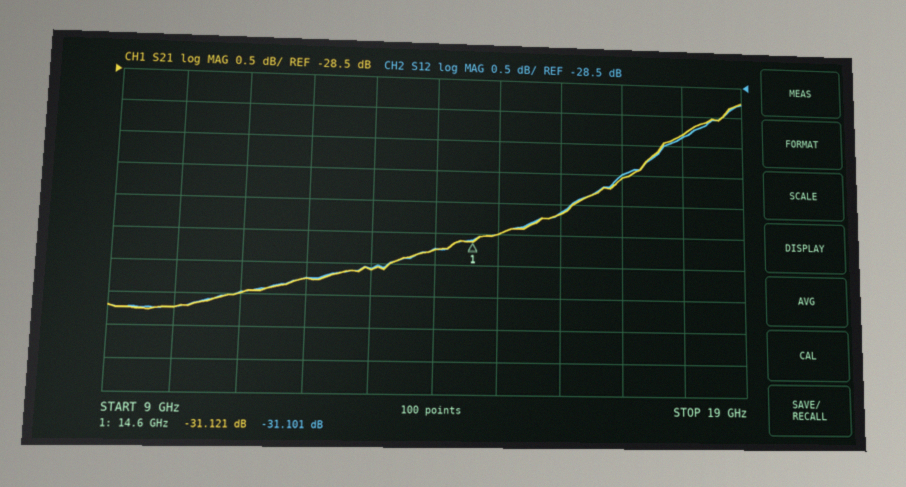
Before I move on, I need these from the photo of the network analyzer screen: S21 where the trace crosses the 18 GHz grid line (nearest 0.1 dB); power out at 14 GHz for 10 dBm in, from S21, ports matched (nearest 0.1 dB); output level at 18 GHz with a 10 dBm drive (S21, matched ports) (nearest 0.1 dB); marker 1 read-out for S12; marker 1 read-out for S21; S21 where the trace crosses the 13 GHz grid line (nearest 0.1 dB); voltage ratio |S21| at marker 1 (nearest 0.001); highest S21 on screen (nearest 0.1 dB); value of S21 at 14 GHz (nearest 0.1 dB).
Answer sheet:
-29.3 dB
-21.3 dBm
-19.3 dBm
-31.101 dB
-31.121 dB
-31.6 dB
0.028
-28.8 dB
-31.3 dB
